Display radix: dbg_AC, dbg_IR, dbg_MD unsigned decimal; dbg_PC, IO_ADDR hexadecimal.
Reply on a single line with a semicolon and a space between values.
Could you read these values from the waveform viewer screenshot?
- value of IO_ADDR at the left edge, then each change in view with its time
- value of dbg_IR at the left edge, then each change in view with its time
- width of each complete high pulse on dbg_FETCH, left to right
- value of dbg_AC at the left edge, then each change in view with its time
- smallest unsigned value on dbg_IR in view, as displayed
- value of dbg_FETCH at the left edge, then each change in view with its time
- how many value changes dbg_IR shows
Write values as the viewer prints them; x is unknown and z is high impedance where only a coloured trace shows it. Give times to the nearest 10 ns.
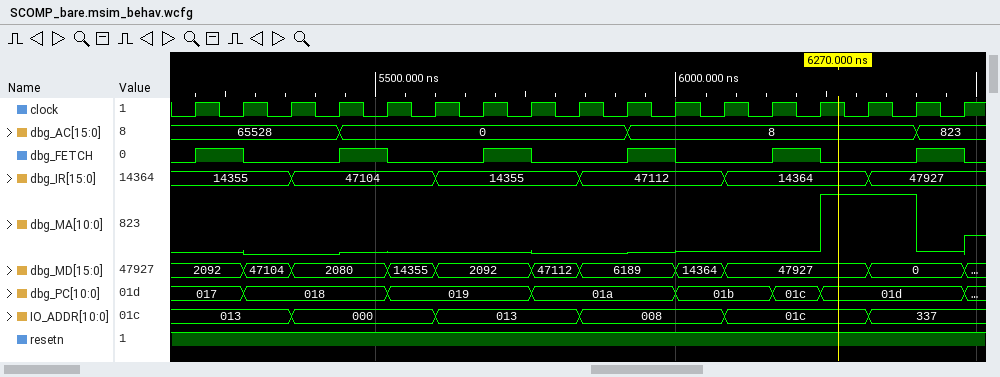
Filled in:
013, 000 at 5360 ns, 013 at 5600 ns, 008 at 5840 ns, 01c at 6080 ns, 337 at 6320 ns; 14355, 47104 at 5360 ns, 14355 at 5600 ns, 47112 at 5840 ns, 14364 at 6080 ns, 47927 at 6320 ns; 80 ns, 80 ns, 80 ns, 80 ns, 80 ns, 80 ns; 65528, 0 at 5440 ns, 8 at 5920 ns, 823 at 6400 ns; 14355; 0, 1 at 5200 ns, 0 at 5280 ns, 1 at 5440 ns, 0 at 5520 ns, 1 at 5680 ns, 0 at 5760 ns, 1 at 5920 ns, 0 at 6000 ns, 1 at 6160 ns, 0 at 6240 ns, 1 at 6400 ns, 0 at 6480 ns; 5
